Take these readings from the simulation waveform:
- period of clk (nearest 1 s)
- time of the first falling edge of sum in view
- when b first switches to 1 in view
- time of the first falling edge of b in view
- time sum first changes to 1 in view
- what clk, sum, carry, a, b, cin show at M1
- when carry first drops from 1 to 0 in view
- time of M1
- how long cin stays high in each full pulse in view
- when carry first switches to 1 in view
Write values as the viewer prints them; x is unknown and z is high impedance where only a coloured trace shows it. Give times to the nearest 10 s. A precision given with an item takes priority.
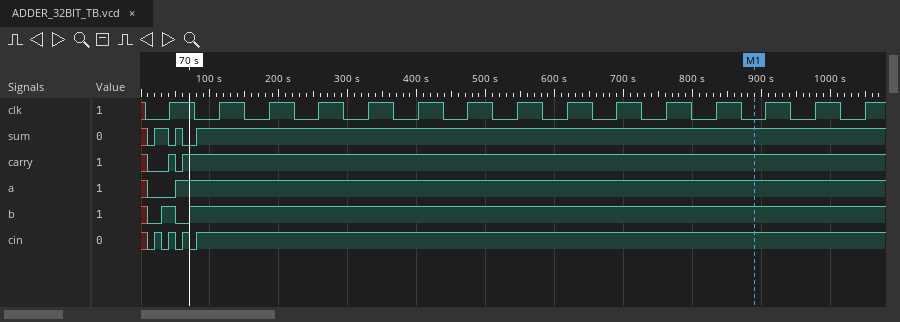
72 s
40 s
30 s
50 s
20 s
clk=0, sum=1, carry=1, a=1, b=1, cin=1
50 s
890 s
10 s, 10 s, 10 s
40 s
